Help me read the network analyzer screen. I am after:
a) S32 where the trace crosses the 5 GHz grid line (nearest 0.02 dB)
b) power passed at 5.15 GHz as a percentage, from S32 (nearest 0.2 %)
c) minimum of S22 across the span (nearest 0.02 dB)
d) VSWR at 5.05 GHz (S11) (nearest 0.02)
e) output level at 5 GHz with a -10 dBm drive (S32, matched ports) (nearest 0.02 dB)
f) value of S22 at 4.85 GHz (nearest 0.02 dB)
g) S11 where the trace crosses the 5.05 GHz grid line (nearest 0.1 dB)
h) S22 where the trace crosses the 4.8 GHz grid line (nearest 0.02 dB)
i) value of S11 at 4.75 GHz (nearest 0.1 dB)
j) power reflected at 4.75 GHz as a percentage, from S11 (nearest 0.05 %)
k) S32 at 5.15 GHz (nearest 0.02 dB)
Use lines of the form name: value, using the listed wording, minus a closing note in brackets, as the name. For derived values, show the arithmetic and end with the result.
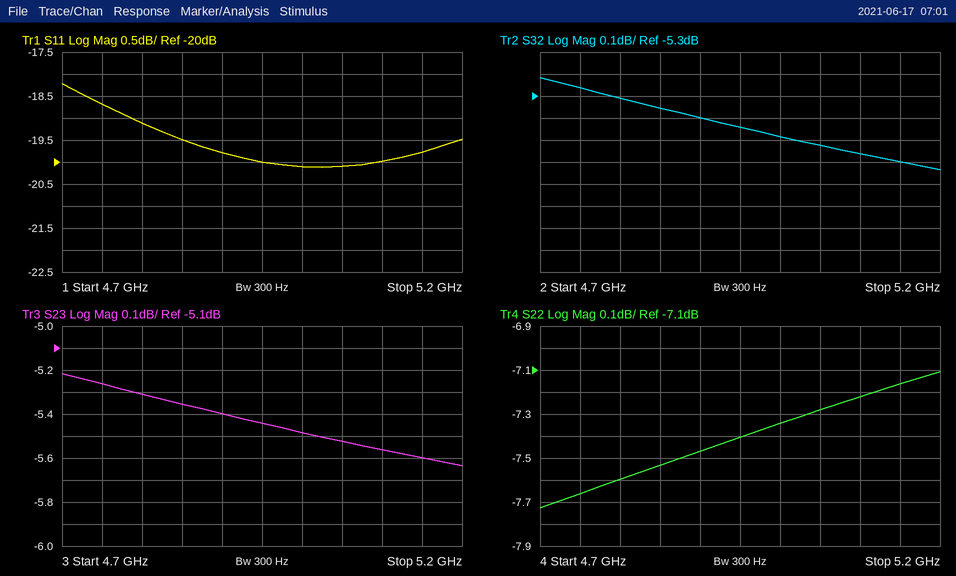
S32 where the trace crosses the 5 GHz grid line: -5.48 dB
power passed at 5.15 GHz as a percentage, from S32: 10^(-5.6/10) ≈ 27.5 %, so 27.6 % to the nearest 0.2 %
minimum of S22 across the span: -7.72 dB
VSWR at 5.05 GHz (S11): |Γ| = 10^(-20.1/20) = 0.0989; VSWR = (1 + 0.0989)/(1 − 0.0989) ≈ 1.22
output level at 5 GHz with a -10 dBm drive (S32, matched ports): -10 dBm + (-5.48 dB) = -15.48 dBm
value of S22 at 4.85 GHz: -7.54 dB
S11 where the trace crosses the 5.05 GHz grid line: -20.1 dB
S22 where the trace crosses the 4.8 GHz grid line: -7.60 dB
value of S11 at 4.75 GHz: -18.7 dB
power reflected at 4.75 GHz as a percentage, from S11: 10^(-18.7/10) ≈ 1.35 %
S32 at 5.15 GHz: -5.60 dB
